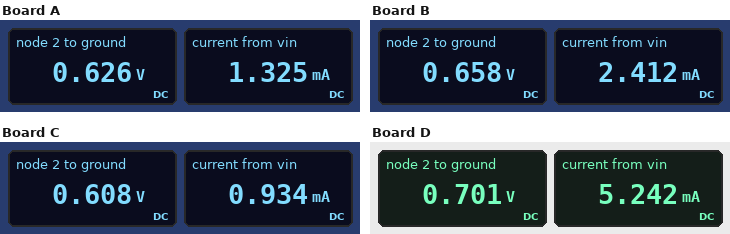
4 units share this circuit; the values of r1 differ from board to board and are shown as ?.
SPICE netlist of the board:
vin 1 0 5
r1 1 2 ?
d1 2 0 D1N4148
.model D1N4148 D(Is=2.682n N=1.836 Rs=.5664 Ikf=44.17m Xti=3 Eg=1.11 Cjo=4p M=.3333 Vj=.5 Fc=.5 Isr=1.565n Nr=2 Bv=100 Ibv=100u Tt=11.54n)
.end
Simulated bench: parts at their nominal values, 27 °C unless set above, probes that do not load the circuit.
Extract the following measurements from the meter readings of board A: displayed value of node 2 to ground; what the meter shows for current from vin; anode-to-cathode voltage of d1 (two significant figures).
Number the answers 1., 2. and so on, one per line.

1. 0.626 V
2. 1.325 mA
3. 630 mV
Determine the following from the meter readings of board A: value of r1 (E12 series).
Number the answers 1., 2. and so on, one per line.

1. 3.3 kΩ
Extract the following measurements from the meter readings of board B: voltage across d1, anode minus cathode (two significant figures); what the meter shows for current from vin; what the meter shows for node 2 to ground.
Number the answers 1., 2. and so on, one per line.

1. 660 mV
2. 2.412 mA
3. 0.658 V
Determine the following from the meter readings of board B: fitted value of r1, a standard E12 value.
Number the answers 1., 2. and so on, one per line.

1. 1.8 kΩ
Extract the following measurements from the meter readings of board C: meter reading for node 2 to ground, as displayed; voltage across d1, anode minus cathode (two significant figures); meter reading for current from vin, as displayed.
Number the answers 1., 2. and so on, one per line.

1. 0.608 V
2. 610 mV
3. 0.934 mA
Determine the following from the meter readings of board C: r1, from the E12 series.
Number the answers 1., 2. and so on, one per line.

1. 4.7 kΩ
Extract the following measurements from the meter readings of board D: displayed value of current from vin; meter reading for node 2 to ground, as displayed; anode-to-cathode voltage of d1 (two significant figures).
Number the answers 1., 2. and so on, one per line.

1. 5.242 mA
2. 0.701 V
3. 700 mV
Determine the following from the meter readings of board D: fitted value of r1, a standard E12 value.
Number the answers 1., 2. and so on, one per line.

1. 820 Ω
